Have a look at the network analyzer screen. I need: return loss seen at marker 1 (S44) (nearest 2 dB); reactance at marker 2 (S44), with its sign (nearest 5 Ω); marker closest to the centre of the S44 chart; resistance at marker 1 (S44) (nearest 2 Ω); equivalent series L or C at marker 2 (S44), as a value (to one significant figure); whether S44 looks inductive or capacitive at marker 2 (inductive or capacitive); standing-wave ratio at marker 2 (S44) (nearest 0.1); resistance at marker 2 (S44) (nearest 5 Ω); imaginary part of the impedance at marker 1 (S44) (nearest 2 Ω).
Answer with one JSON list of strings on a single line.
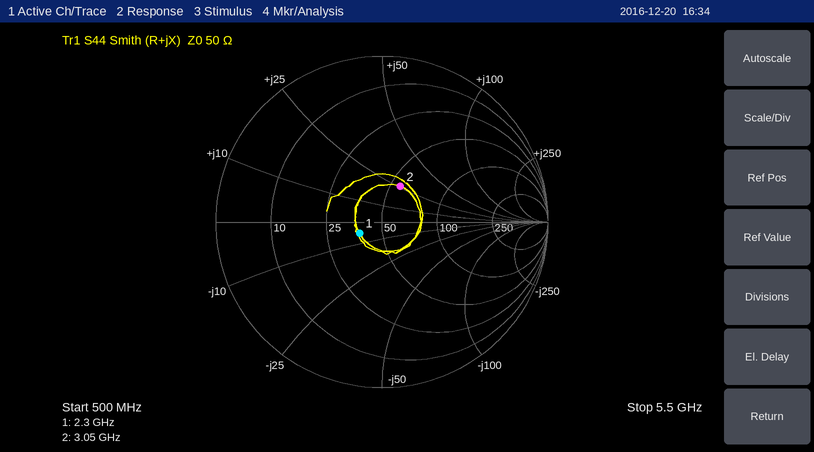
["16 dB", "+25 Ω", "marker 1", "38 Ω", "1 nH", "inductive", "1.6", "55 Ω", "-6 Ω"]
